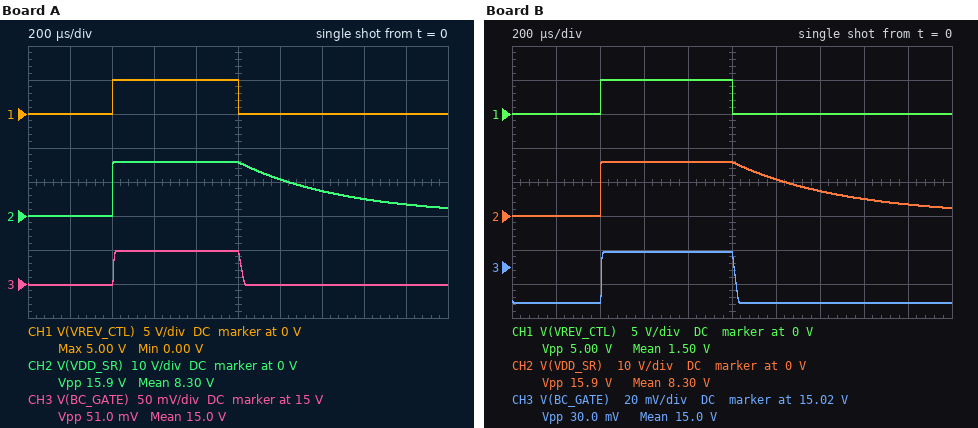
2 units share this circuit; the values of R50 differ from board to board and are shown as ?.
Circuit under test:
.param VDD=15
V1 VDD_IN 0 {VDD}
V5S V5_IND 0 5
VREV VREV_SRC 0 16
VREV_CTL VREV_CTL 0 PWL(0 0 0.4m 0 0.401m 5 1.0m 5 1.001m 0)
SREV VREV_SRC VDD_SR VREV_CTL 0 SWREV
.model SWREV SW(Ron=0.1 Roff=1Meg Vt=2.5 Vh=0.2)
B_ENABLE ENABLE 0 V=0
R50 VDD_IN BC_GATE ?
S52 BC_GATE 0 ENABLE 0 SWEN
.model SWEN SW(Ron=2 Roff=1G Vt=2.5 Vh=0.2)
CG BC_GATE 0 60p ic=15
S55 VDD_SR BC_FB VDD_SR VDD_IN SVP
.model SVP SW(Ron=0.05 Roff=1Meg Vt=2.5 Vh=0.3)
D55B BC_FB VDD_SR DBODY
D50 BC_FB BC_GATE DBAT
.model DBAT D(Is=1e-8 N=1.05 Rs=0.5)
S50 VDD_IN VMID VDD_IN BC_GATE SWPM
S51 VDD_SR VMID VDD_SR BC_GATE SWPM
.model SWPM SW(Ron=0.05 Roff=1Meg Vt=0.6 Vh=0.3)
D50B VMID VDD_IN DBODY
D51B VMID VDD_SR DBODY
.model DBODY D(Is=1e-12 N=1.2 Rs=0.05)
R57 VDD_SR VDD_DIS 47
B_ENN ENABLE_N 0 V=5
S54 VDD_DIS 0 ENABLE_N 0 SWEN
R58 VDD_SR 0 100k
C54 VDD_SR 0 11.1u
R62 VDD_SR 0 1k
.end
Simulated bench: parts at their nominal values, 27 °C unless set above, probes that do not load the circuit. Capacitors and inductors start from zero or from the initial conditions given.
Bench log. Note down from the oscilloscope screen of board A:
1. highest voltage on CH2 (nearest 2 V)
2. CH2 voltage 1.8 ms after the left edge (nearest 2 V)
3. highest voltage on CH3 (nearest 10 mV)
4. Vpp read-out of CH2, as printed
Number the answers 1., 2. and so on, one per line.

1. 16 V
2. 4 V
3. 15.05 V
4. 15.9 V
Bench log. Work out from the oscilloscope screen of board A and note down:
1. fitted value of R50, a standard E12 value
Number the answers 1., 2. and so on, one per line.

1. 68 kΩ
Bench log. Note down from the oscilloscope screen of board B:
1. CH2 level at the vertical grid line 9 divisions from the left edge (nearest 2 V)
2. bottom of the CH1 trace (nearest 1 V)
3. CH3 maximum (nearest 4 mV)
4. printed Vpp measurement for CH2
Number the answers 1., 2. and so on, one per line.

1. 4 V
2. 0 V
3. 15.028 V
4. 15.9 V
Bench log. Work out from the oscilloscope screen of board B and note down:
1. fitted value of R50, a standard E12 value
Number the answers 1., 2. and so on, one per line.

1. 39 kΩ
